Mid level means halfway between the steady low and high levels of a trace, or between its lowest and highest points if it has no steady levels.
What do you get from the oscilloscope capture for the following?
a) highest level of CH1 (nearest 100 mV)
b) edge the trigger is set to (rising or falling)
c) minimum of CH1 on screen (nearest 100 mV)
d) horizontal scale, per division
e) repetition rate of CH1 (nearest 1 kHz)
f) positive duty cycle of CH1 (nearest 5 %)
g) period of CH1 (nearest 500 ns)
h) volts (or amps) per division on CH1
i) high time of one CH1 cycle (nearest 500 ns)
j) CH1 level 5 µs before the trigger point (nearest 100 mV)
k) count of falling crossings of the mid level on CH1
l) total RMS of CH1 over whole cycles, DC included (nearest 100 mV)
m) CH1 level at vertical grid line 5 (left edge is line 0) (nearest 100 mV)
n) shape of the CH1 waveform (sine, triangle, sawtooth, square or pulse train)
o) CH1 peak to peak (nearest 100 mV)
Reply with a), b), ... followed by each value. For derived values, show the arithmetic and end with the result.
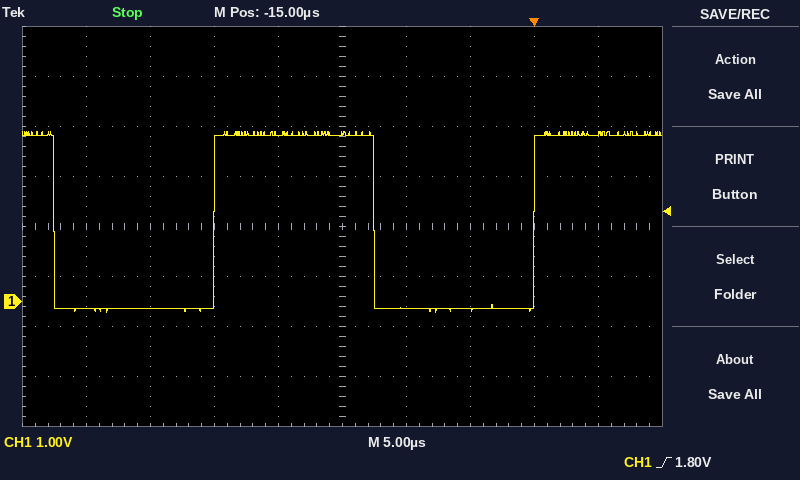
a) 3.4 V
b) rising
c) -200 mV
d) 5 µs
e) 1 / 25.0 µs ≈ 40 kHz
f) 12.5 µs / 25.0 µs ≈ 50 %
g) 25.0 µs
h) 1 V
i) 12.5 µs
j) -200 mV
k) 2
l) √(0.5 × (3.4 V)² + 0.5 × (-200 mV)²) ≈ 2.4 V
m) 3.4 V
n) square
o) 3.4 V − (-200 mV) = 3.6 V
